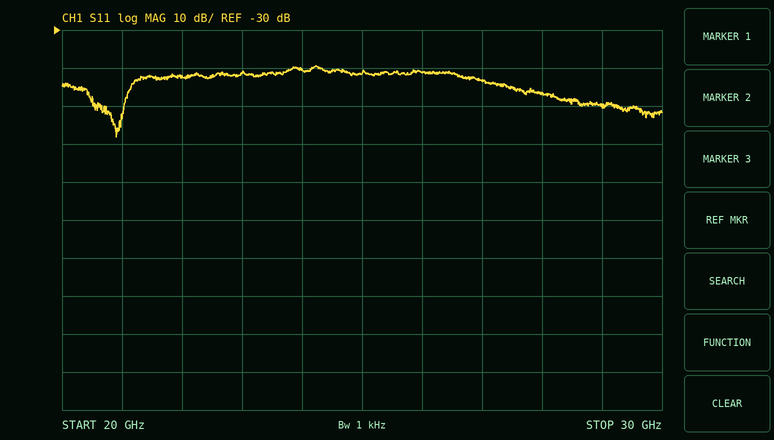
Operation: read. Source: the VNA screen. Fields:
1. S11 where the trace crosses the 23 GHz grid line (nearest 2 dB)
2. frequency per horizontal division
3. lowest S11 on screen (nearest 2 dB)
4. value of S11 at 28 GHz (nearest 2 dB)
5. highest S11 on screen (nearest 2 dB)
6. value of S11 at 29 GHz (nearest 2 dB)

-42 dB
1 GHz
-58 dB
-46 dB
-40 dB
-50 dB
